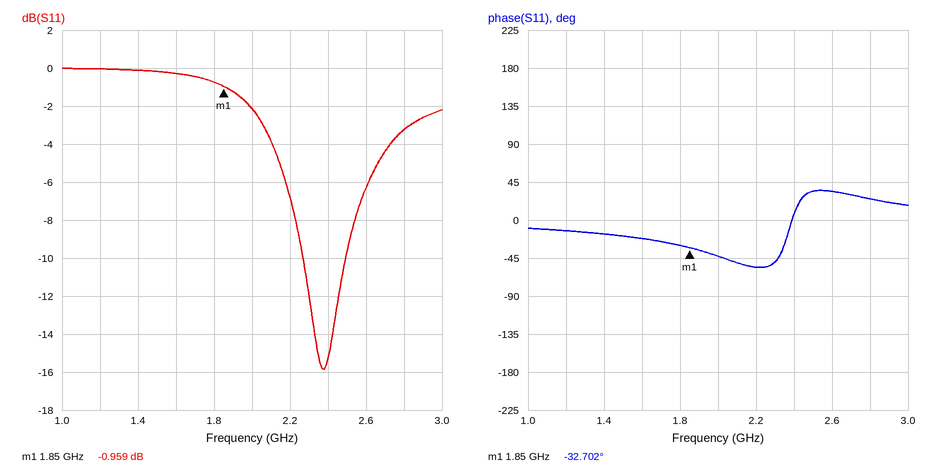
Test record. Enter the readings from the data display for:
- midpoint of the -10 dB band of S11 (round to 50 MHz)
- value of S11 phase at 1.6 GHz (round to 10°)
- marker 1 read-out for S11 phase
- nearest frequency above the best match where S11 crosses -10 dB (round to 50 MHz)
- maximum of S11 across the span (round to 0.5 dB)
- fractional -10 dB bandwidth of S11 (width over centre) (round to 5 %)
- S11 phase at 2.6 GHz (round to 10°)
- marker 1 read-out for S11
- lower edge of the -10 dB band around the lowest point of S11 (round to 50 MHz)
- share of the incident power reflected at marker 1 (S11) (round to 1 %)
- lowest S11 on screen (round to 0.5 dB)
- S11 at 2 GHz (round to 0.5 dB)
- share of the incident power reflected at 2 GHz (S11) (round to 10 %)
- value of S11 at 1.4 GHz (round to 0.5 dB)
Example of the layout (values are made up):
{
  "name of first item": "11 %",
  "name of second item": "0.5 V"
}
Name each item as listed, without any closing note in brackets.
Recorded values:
{
  "midpoint of the -10 dB band of S11": "2.40 GHz",
  "value of S11 phase at 1.6 GHz": "-20°",
  "marker 1 read-out for S11 phase": "-32.702°",
  "nearest frequency above the best match where S11 crosses -10 dB": "2.50 GHz",
  "maximum of S11 across the span": "0.0 dB",
  "fractional -10 dB bandwidth of S11 (width over centre)": "10 %",
  "S11 phase at 2.6 GHz": "30°",
  "marker 1 read-out for S11": "-0.959 dB",
  "lower edge of the -10 dB band around the lowest point of S11": "2.25 GHz",
  "share of the incident power reflected at marker 1 (S11)": "80 %",
  "lowest S11 on screen": "-16.0 dB",
  "S11 at 2 GHz": "-2.0 dB",
  "share of the incident power reflected at 2 GHz (S11)": "60 %",
  "value of S11 at 1.4 GHz": "0.0 dB"
}
